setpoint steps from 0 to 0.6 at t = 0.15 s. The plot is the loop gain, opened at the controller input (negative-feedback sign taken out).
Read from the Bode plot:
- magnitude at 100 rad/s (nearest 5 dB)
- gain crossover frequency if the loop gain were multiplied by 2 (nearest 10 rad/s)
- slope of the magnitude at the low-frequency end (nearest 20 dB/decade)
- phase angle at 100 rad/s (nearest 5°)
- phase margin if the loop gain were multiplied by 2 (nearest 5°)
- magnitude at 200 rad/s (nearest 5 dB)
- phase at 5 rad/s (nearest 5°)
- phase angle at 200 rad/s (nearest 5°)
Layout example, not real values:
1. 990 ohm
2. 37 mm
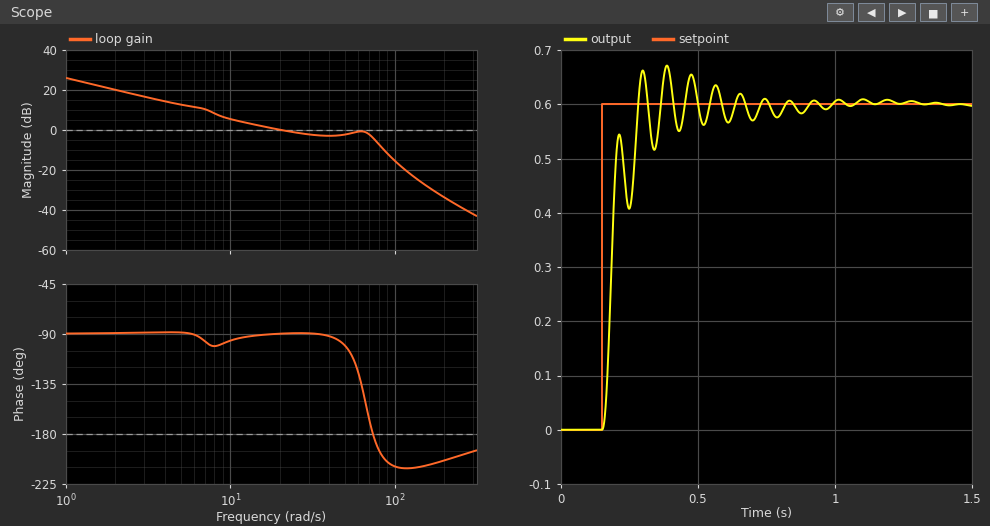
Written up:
1. -15 dB
2. 80 rad/s
3. -20 dB/decade
4. -210°
5. -10°
6. -35 dB
7. -90°
8. -205°
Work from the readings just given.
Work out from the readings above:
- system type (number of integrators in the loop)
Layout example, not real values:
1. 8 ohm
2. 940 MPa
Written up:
1. 1
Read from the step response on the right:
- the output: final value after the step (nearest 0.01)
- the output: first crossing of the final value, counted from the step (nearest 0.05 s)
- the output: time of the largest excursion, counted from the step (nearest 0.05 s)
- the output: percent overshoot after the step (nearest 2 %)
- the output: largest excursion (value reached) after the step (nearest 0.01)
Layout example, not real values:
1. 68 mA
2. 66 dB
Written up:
1. 0.60
2. 0.15 s
3. 0.25 s
4. 12 %
5. 0.67
